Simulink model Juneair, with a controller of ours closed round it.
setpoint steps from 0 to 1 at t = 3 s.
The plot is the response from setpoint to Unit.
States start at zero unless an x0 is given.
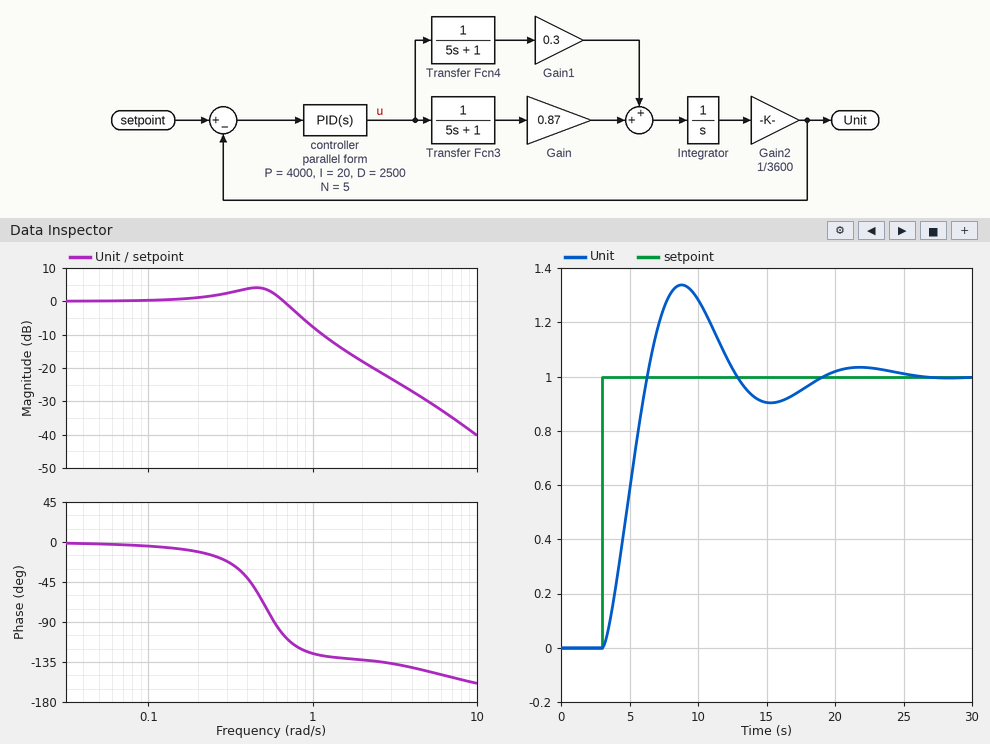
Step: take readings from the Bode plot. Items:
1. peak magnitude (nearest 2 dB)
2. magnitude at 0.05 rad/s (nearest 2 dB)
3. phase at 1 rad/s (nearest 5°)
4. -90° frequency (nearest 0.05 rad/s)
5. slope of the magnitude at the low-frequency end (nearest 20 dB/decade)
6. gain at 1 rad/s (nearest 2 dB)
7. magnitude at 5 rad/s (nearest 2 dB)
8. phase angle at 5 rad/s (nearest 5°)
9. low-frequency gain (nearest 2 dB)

4 dB
0 dB
-125°
0.60 rad/s
0 dB/decade
-8 dB
-30 dB
-145°
0 dB
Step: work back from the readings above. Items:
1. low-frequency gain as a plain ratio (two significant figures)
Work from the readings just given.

1.0
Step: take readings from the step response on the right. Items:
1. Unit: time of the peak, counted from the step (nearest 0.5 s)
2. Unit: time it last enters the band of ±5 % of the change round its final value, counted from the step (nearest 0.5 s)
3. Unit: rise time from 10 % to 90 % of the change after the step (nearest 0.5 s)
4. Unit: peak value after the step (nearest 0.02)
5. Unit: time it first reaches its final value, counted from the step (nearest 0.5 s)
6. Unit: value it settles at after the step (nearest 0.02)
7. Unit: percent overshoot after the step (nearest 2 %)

6.0 s
14.5 s
2.5 s
1.34
3.5 s
1.00
34 %
